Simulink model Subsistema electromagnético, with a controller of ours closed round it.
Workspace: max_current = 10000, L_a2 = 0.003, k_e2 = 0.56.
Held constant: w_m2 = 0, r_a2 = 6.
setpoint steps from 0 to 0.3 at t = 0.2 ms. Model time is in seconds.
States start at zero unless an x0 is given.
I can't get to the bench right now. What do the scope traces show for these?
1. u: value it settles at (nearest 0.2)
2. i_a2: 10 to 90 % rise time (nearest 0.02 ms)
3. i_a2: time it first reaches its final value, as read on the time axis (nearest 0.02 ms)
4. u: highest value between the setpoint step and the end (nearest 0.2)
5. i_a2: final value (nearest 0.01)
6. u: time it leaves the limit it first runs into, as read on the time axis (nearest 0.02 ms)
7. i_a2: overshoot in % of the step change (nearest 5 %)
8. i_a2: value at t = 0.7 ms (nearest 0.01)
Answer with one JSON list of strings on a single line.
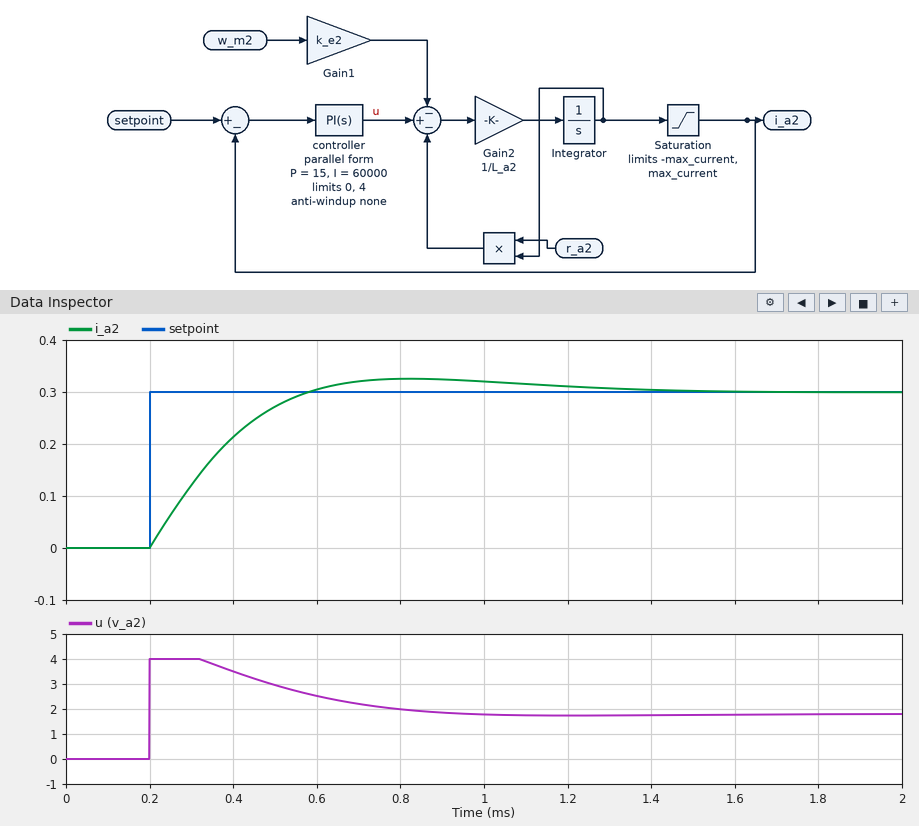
["1.8", "0.28 ms", "0.58 ms", "4.0", "0.30", "0.32 ms", "10 %", "0.32"]
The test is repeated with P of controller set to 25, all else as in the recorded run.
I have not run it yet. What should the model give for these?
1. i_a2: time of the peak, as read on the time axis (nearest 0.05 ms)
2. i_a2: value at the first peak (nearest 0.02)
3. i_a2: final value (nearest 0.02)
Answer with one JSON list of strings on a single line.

["0.75 ms", "0.32", "0.30"]
